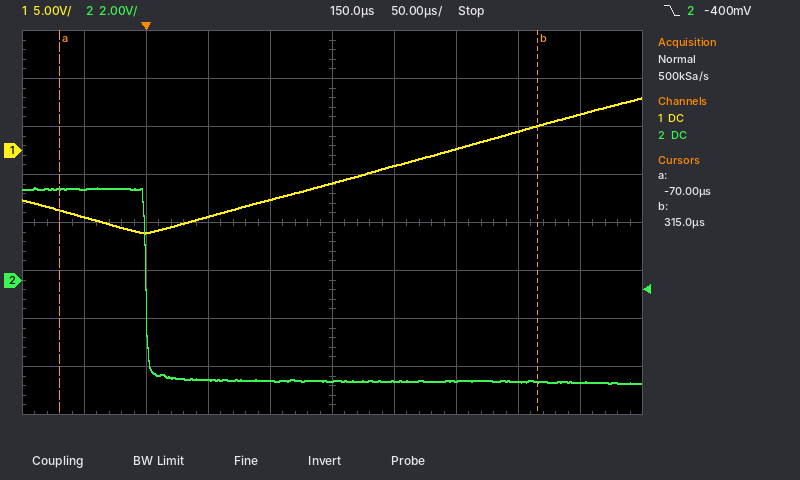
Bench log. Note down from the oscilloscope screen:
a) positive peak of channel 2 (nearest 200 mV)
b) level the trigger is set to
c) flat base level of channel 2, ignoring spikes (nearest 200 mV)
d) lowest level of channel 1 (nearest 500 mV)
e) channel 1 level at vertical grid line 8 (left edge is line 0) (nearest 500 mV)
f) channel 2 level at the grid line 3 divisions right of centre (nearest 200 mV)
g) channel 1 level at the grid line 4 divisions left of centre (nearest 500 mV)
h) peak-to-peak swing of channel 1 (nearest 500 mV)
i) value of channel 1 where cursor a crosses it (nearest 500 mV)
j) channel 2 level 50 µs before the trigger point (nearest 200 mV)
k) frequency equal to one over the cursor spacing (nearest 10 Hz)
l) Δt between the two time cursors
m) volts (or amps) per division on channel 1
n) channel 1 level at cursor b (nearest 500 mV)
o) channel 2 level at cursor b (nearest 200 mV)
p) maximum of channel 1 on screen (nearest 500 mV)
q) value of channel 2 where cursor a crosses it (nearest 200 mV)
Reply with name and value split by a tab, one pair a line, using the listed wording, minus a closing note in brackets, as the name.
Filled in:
positive peak of channel 2	3.8 V
level the trigger is set to	-400 mV
flat base level of channel 2, ignoring spikes	-4.2 V
lowest level of channel 1	-8.5 V
channel 1 level at vertical grid line 8 (left edge is line 0)	2.0 V
channel 2 level at the grid line 3 divisions right of centre	-4.2 V
channel 1 level at the grid line 4 divisions left of centre	-7.0 V
peak-to-peak swing of channel 1	14.0 V
value of channel 1 where cursor a crosses it	-6.0 V
channel 2 level 50 µs before the trigger point	3.8 V
frequency equal to one over the cursor spacing	2.60 kHz
Δt between the two time cursors	385 µs
volts (or amps) per division on channel 1	5 V
channel 1 level at cursor b	2.5 V
channel 2 level at cursor b	-4.2 V
maximum of channel 1 on screen	5.5 V
value of channel 2 where cursor a crosses it	3.8 V
